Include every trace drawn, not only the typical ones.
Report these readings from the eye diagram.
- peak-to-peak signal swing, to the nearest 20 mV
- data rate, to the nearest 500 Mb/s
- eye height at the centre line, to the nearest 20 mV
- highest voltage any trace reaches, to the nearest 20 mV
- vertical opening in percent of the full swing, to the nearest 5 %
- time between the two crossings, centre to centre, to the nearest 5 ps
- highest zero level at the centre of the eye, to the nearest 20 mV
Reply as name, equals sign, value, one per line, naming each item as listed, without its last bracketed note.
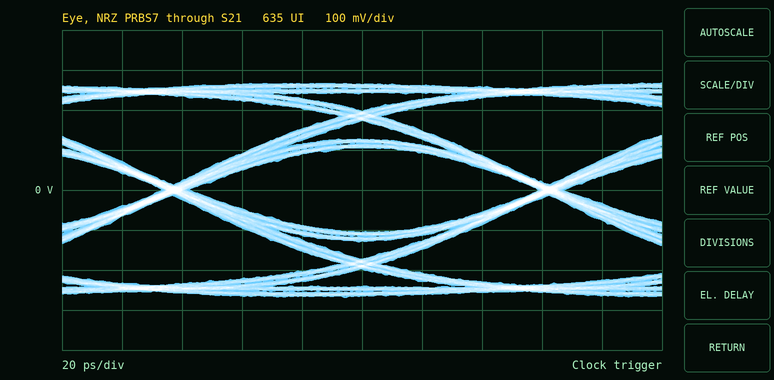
peak-to-peak signal swing, to the nearest 20 mV = 540 mV
data rate, to the nearest 500 Mb/s = 8.0 Gb/s
eye height at the centre line, to the nearest 20 mV = 220 mV
highest voltage any trace reaches, to the nearest 20 mV = 260 mV
vertical opening in percent of the full swing, to the nearest 5 % = 40 %
time between the two crossings, centre to centre, to the nearest 5 ps = 125 ps
highest zero level at the centre of the eye, to the nearest 20 mV = -100 mV
